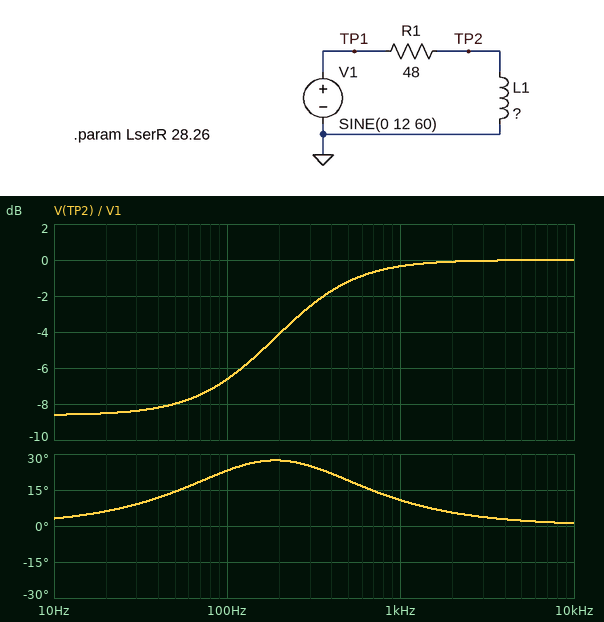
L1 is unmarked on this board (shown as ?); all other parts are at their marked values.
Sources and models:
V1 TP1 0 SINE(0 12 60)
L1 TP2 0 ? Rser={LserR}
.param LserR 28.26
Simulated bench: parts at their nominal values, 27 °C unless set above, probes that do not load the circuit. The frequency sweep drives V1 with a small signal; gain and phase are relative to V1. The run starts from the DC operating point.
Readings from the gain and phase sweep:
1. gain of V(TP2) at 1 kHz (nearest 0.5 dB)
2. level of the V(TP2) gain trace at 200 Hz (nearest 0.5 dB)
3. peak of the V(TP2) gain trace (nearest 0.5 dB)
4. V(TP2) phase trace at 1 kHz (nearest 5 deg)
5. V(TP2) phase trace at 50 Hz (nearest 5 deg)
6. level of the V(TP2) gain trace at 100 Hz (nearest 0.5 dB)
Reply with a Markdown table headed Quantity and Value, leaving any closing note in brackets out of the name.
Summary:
| Quantity | Value |
|---|---|
| gain of V(TP2) at 1 kHz | -0.5 dB |
| level of the V(TP2) gain trace at 200 Hz | -4.0 dB |
| peak of the V(TP2) gain trace | 0 dB |
| V(TP2) phase trace at 1 kHz | 10 deg |
| V(TP2) phase trace at 50 Hz | 15 deg |
| level of the V(TP2) gain trace at 100 Hz | -6.5 dB |
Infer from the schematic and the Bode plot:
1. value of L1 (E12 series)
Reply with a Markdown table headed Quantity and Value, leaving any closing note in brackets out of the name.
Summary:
| Quantity | Value |
|---|---|
| value of L1 | 39 mH |
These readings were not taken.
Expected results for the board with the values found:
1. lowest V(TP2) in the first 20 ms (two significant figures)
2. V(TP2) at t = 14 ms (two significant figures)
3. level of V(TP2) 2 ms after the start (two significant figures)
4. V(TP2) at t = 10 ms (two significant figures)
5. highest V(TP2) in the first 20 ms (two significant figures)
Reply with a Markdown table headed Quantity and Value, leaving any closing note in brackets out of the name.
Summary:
| Quantity | Value |
|---|---|
| lowest V(TP2) in the first 20 ms | -4.9 V |
| V(TP2) at t = 14 ms | -3.2 V |
| level of V(TP2) 2 ms after the start | 4.2 V |
| V(TP2) at t = 10 ms | -3.9 V |
| highest V(TP2) in the first 20 ms | 4.9 V |
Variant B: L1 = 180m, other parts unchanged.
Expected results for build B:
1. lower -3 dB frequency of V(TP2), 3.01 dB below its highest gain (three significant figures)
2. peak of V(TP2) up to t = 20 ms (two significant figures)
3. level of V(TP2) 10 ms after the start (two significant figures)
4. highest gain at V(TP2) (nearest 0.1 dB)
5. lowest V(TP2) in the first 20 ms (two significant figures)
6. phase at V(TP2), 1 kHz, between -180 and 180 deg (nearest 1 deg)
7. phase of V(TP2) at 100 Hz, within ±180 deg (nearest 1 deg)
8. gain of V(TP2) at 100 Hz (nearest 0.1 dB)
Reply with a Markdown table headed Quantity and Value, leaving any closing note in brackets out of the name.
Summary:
| Quantity | Value |
|---|---|
| lower -3 dB frequency of V(TP2), 3.01 dB below its highest gain | 57.4 Hz |
| peak of V(TP2) up to t = 20 ms | 8.6 V |
| level of V(TP2) 10 ms after the start | -7.7 V |
| highest gain at V(TP2) | 0 dB |
| lowest V(TP2) in the first 20 ms | -8.7 V |
| phase at V(TP2), 1 kHz, between -180 and 180 deg | 2 deg |
| phase of V(TP2) at 100 Hz, within ±180 deg | 20 deg |
| gain of V(TP2) at 100 Hz | -1.4 dB |
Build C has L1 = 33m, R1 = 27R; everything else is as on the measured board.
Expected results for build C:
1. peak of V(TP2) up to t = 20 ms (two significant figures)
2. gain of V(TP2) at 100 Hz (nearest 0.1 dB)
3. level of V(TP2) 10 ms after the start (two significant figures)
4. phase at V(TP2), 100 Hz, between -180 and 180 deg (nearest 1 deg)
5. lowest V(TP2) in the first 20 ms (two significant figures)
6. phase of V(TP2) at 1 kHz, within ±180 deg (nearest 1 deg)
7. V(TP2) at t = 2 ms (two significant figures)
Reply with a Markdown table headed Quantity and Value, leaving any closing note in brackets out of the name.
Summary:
| Quantity | Value |
|---|---|
| peak of V(TP2) up to t = 20 ms | 6.5 V |
| gain of V(TP2) at 100 Hz | -4.5 dB |
| level of V(TP2) 10 ms after the start | -4.8 V |
| phase at V(TP2), 100 Hz, between -180 and 180 deg | 16 deg |
| lowest V(TP2) in the first 20 ms | -6.5 V |
| phase of V(TP2) at 1 kHz, within ±180 deg | 7 deg |
| V(TP2) at t = 2 ms | 5.3 V |
